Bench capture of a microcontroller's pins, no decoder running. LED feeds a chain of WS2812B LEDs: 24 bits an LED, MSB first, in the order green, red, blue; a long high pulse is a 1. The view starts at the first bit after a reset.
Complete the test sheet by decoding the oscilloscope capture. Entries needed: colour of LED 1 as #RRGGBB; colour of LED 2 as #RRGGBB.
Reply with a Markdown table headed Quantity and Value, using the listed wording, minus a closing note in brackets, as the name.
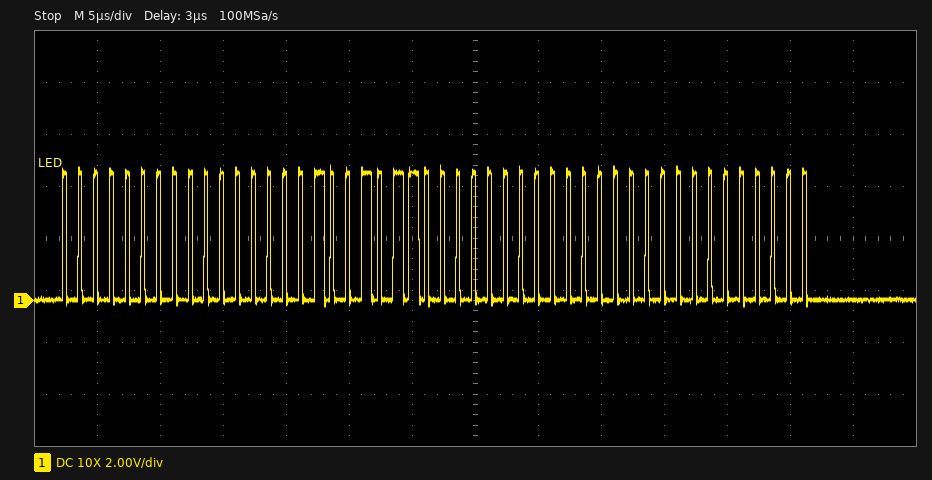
| Quantity | Value |
|---|---|
| colour of LED 1 as #RRGGBB | #000096 |
| colour of LED 2 as #RRGGBB | #000000 |
